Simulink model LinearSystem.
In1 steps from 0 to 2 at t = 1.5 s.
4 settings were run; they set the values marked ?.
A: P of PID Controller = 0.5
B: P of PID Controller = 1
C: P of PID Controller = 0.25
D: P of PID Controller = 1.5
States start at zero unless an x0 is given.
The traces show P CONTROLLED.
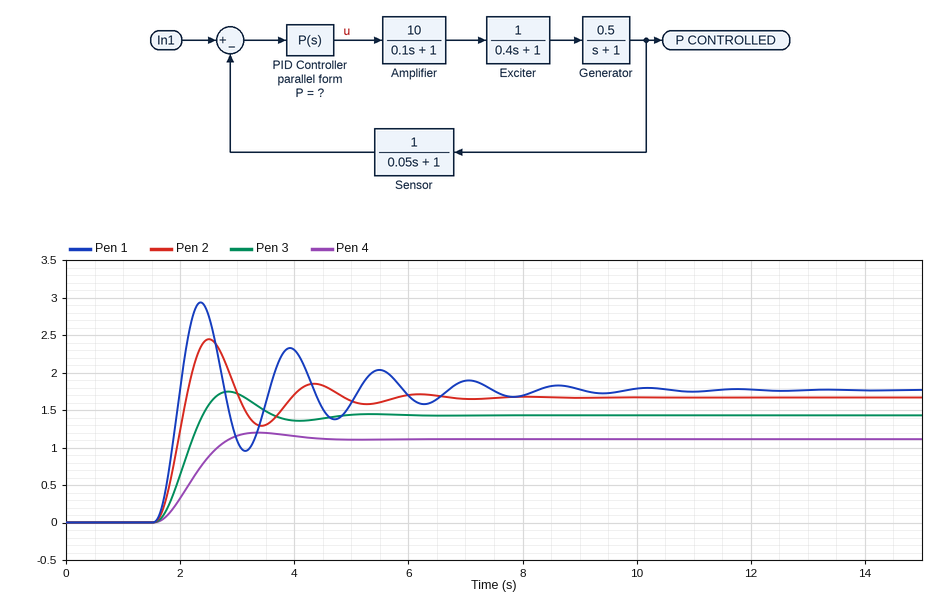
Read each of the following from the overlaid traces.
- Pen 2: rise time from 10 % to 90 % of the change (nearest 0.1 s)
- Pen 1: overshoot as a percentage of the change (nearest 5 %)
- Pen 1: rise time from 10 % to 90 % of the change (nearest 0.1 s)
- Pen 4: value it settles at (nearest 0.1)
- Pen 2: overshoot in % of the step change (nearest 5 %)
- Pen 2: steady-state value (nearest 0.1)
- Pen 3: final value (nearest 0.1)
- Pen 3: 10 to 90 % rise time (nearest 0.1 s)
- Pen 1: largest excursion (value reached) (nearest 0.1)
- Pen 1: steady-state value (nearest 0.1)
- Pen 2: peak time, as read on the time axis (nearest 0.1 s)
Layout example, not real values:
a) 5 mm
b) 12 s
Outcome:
a) 0.4 s
b) 65 %
c) 0.3 s
d) 1.1
e) 45 %
f) 1.7
g) 1.4
h) 0.6 s
i) 2.9
j) 1.8
k) 2.5 s
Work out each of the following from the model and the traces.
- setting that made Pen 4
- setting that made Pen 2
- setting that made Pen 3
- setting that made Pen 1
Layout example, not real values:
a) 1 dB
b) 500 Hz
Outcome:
a) C
b) B
c) A
d) D
